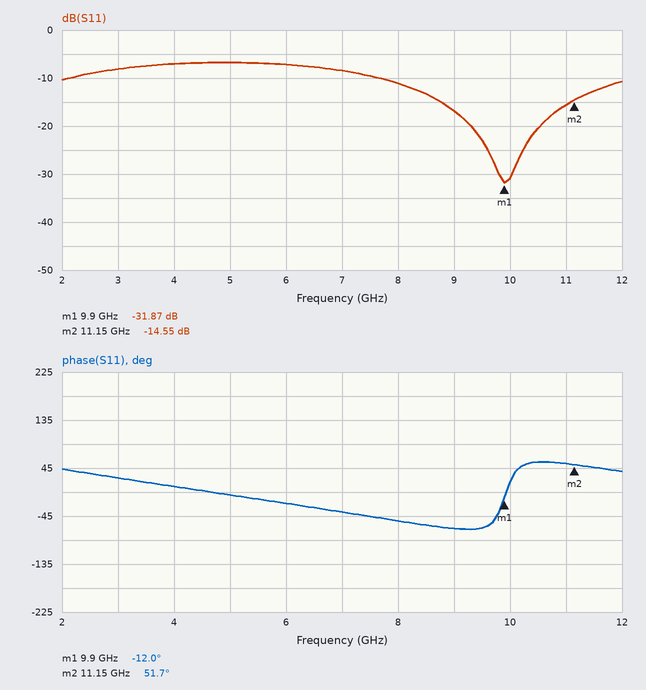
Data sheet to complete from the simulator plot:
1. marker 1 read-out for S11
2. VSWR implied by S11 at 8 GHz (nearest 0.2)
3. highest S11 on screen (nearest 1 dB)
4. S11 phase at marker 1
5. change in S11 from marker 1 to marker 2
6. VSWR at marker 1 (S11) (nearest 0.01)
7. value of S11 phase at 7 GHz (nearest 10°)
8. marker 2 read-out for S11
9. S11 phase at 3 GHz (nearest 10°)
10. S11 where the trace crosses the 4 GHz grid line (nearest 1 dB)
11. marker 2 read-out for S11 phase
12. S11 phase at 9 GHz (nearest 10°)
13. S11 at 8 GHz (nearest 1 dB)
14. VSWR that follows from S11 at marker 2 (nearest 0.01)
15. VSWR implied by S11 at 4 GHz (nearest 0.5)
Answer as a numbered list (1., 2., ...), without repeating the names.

1. -31.87 dB
2. 1.8
3. -7 dB
4. -12.0°
5. 17.32 dB
6. 1.05
7. -40°
8. -14.55 dB
9. 30°
10. -7 dB
11. 51.7°
12. -70°
13. -11 dB
14. 1.46
15. 2.5
